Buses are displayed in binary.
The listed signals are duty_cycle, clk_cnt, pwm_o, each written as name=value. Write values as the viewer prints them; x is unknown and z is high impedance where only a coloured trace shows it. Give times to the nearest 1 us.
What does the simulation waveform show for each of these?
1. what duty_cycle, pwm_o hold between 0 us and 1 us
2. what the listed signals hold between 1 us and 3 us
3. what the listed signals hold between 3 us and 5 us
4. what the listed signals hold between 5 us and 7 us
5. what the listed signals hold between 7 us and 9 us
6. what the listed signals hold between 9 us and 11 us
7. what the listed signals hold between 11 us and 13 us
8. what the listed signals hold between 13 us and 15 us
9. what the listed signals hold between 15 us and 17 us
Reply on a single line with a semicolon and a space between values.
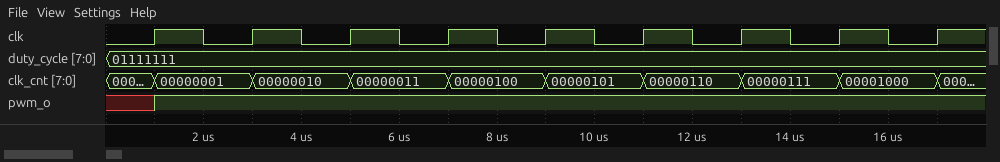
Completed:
duty_cycle=01111111, pwm_o=x; duty_cycle=01111111, clk_cnt=00000001, pwm_o=1; duty_cycle=01111111, clk_cnt=00000010, pwm_o=1; duty_cycle=01111111, clk_cnt=00000011, pwm_o=1; duty_cycle=01111111, clk_cnt=00000100, pwm_o=1; duty_cycle=01111111, clk_cnt=00000101, pwm_o=1; duty_cycle=01111111, clk_cnt=00000110, pwm_o=1; duty_cycle=01111111, clk_cnt=00000111, pwm_o=1; duty_cycle=01111111, clk_cnt=00001000, pwm_o=1
